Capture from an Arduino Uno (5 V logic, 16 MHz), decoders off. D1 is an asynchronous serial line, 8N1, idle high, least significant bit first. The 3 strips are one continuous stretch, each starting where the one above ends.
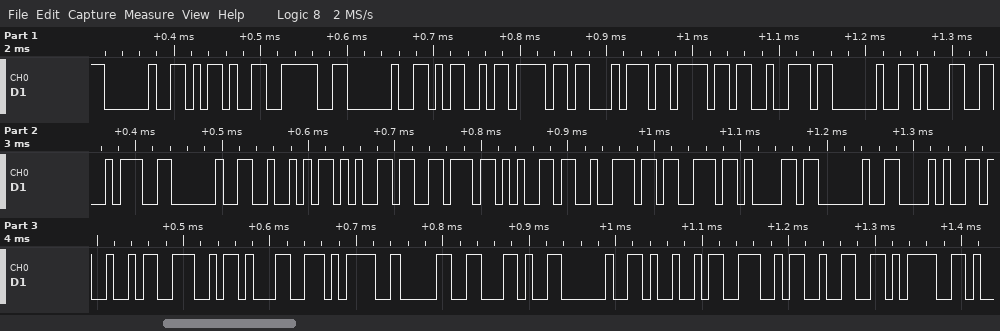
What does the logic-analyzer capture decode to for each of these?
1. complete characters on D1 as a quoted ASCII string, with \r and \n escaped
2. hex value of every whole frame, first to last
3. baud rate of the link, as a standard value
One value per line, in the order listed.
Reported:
" -> Motor 1: Reversa (IN1=0, IN2="
0x20 0x2D 0x3E 0x20 0x4D 0x6F 0x74 0x6F 0x72 0x20 0x31 0x3A 0x20 0x52 0x65 0x76 0x65 0x72 0x73 0x61 0x20 0x28 0x49 0x4E 0x31 0x3D 0x30 0x2C 0x20 0x49 0x4E 0x32 0x3D
115200 baud
